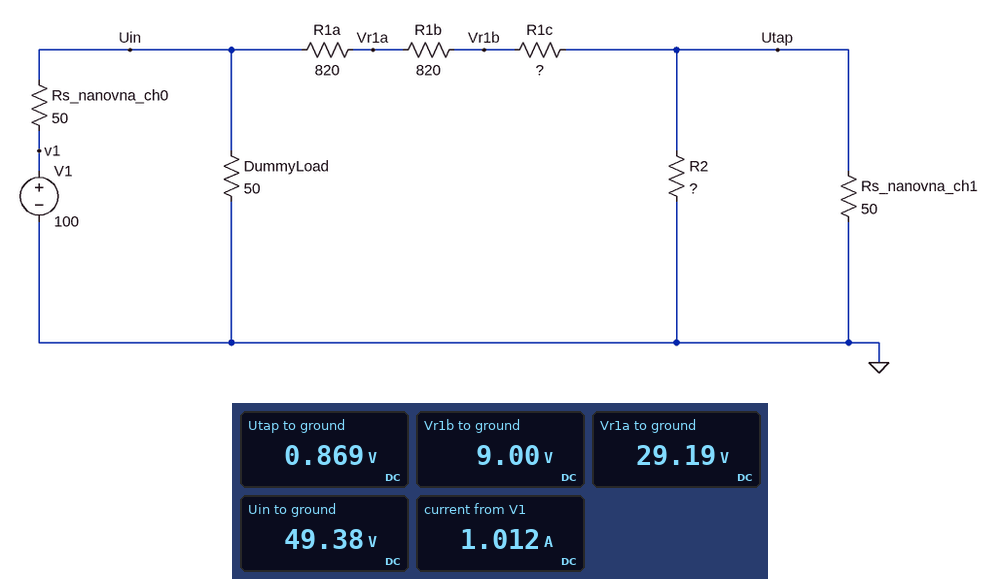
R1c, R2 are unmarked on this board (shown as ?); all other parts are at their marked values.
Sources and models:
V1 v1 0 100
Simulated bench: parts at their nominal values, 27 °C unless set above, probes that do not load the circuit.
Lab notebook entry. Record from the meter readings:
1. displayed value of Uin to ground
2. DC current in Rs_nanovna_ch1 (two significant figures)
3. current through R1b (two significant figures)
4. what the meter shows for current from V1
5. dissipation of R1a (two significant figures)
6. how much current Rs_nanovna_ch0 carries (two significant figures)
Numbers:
49.38 V
17 mA
25 mA
1.012 A
500 mW
1.0 A
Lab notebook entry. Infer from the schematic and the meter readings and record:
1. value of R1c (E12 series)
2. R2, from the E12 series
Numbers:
330 Ω
120 Ω
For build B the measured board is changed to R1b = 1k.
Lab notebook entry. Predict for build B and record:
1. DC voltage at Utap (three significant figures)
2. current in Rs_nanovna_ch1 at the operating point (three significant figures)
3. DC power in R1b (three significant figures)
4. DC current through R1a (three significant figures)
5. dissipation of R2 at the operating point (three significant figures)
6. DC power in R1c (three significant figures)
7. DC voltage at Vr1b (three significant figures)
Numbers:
798 mV
16.0 mA
512 mW
22.6 mA
5.31 mW
169 mW
8.26 V
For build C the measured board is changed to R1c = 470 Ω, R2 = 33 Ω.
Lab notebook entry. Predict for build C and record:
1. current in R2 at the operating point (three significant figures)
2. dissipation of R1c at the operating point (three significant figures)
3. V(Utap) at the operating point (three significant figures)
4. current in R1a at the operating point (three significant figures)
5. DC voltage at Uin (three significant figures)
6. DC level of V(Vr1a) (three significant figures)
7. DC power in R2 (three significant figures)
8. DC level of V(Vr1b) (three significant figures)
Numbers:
14.0 mA
253 mW
461 mV
23.2 mA
49.4 V
30.4 V
6.45 mW
11.4 V
